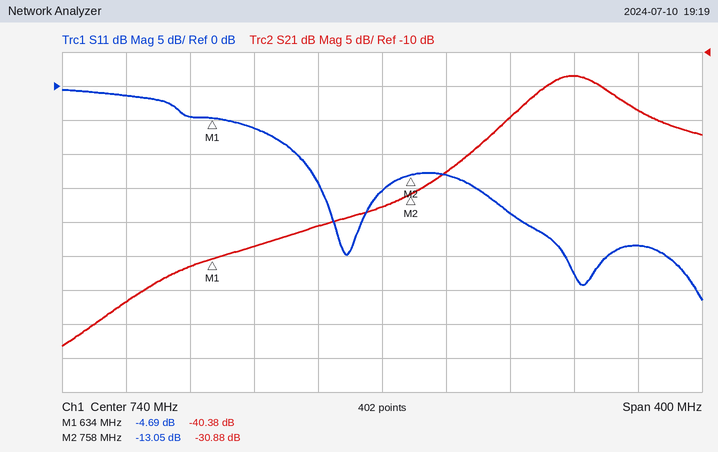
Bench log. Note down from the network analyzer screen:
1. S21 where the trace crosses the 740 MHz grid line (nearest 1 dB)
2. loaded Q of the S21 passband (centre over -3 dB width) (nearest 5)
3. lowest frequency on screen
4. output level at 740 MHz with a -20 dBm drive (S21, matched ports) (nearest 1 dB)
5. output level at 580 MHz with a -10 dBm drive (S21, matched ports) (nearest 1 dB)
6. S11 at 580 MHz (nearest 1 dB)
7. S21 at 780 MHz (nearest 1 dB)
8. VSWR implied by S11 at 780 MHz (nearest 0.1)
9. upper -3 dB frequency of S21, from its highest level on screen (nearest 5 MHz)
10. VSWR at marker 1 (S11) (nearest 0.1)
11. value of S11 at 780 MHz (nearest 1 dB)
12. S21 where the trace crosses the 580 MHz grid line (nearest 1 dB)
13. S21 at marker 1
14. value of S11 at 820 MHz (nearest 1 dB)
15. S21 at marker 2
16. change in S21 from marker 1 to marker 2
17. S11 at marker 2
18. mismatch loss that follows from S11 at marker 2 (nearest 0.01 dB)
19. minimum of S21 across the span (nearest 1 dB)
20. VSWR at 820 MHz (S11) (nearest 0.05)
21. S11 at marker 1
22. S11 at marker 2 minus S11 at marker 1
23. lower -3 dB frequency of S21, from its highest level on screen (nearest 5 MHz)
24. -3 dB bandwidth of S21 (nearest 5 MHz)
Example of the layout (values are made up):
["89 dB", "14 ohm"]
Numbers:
["-33 dB", "15", "540 MHz", "-53 dBm", "-57 dBm", "-1 dB", "-28 dB", "1.6", "885 MHz", "3.8", "-13 dB", "-47 dB", "-40.38 dB", "-19 dB", "-30.88 dB", "9.50 dB", "-13.05 dB", "0.22 dB", "-53 dB", "1.25", "-4.69 dB", "-8.36 dB", "835 MHz", "50 MHz"]
